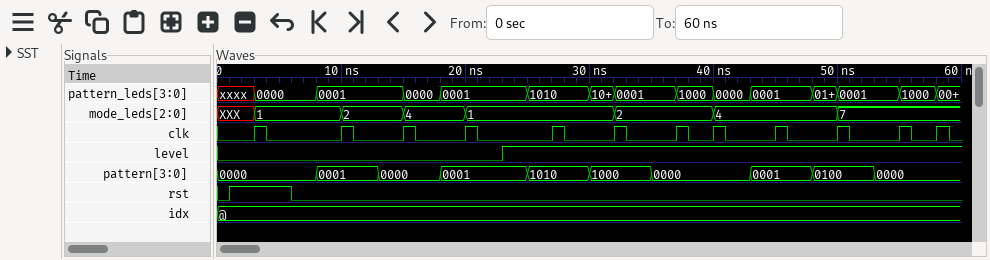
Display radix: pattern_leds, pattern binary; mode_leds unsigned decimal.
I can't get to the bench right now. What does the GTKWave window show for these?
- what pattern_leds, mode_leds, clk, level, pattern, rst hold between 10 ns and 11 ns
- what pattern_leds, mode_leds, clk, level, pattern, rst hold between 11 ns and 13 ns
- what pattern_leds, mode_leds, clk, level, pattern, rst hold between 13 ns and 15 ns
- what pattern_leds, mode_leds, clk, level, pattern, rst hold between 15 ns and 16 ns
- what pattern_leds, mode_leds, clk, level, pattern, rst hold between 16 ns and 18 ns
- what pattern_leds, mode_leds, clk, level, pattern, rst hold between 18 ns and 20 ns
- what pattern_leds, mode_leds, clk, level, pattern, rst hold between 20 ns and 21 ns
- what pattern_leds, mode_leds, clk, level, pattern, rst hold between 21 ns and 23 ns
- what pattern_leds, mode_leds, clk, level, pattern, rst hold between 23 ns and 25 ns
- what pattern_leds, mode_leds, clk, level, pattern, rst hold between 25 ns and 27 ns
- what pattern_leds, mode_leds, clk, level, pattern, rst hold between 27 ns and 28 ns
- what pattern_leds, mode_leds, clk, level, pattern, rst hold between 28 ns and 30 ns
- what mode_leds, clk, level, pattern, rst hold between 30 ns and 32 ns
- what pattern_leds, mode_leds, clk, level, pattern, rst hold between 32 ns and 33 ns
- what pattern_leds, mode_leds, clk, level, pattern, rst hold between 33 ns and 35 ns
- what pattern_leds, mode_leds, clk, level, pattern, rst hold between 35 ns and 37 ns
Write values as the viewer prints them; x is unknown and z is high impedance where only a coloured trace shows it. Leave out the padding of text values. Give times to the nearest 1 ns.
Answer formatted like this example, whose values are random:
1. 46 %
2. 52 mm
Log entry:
1. pattern_leds=0001, mode_leds=2, clk=1, level=0, pattern=0001, rst=0
2. pattern_leds=0001, mode_leds=2, clk=0, level=0, pattern=0001, rst=0
3. pattern_leds=0001, mode_leds=2, clk=0, level=0, pattern=0000, rst=0
4. pattern_leds=0000, mode_leds=4, clk=1, level=0, pattern=0000, rst=0
5. pattern_leds=0000, mode_leds=4, clk=0, level=0, pattern=0000, rst=0
6. pattern_leds=0001, mode_leds=4, clk=0, level=0, pattern=0001, rst=0
7. pattern_leds=0001, mode_leds=1, clk=1, level=0, pattern=0001, rst=0
8. pattern_leds=0001, mode_leds=1, clk=0, level=0, pattern=0001, rst=0
9. pattern_leds=0001, mode_leds=1, clk=0, level=1, pattern=0001, rst=0
10. pattern_leds=1010, mode_leds=1, clk=0, level=1, pattern=1010, rst=0
11. pattern_leds=1010, mode_leds=1, clk=1, level=1, pattern=1010, rst=0
12. pattern_leds=1010, mode_leds=1, clk=0, level=1, pattern=1010, rst=0
13. mode_leds=1, clk=0, level=1, pattern=1000, rst=0
14. pattern_leds=0001, mode_leds=2, clk=1, level=1, pattern=1000, rst=0
15. pattern_leds=0001, mode_leds=2, clk=0, level=1, pattern=1000, rst=0
16. pattern_leds=0001, mode_leds=2, clk=0, level=1, pattern=0000, rst=0
